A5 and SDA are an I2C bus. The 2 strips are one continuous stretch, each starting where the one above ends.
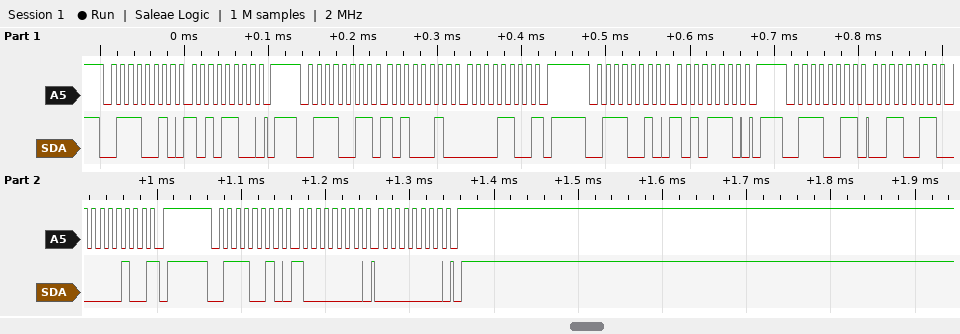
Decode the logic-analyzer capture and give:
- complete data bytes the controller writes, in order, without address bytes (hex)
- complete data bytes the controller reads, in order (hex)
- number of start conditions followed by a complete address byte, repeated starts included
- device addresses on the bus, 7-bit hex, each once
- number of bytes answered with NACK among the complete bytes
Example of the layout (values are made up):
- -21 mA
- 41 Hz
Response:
- AC AE 80 00
- A2 0C 33 04
- 5
- 0x39
- 2
